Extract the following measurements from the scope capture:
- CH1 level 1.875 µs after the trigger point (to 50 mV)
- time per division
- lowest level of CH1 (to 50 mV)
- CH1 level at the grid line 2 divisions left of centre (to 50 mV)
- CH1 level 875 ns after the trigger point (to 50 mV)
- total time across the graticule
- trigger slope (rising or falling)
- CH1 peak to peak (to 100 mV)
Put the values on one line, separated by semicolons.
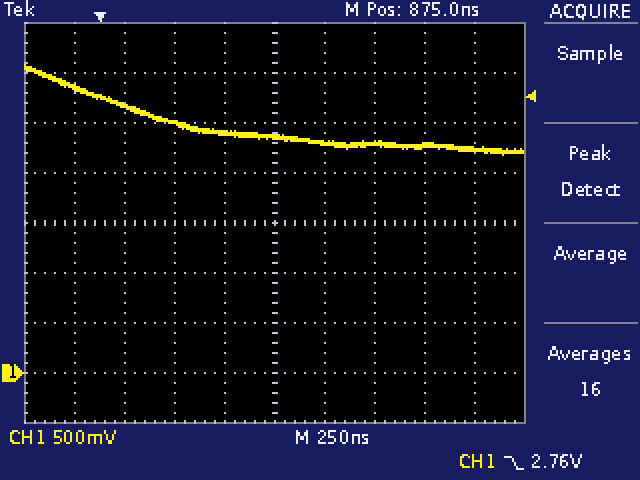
2.25 V; 250 ns; 2.20 V; 2.50 V; 2.35 V; 2.5 µs; falling; 900 mV
